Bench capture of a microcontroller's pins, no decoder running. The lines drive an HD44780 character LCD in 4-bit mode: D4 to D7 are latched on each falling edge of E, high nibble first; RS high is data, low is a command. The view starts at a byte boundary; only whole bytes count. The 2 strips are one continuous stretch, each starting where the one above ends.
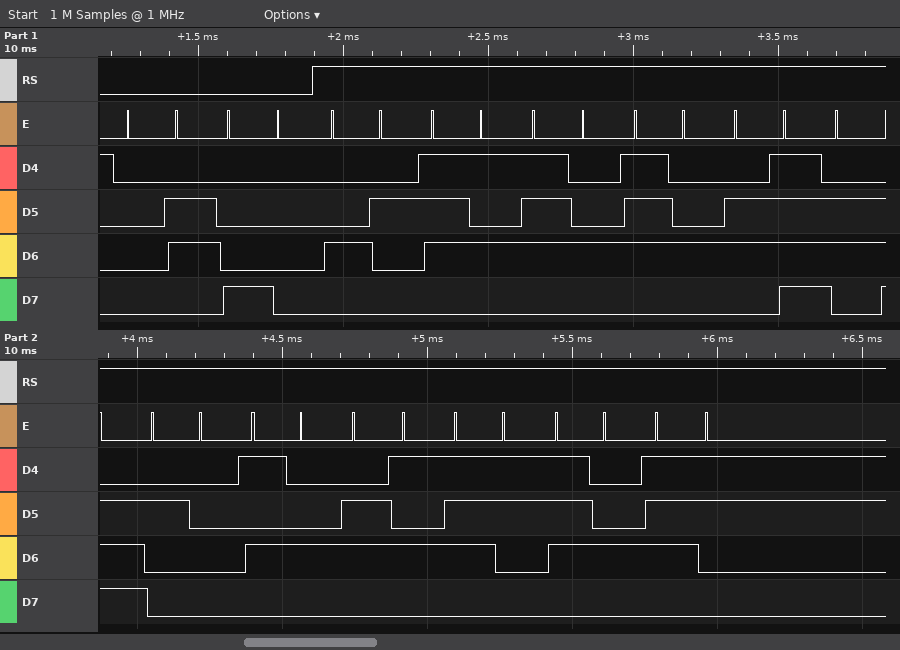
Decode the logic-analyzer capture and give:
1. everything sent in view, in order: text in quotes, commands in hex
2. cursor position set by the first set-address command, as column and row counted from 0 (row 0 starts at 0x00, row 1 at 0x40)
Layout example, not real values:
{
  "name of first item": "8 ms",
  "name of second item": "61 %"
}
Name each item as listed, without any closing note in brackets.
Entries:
{
  "everything sent in view, in order: text in quotes, commands in hex": "0x06 0x80 \"Button Tests\"",
  "cursor position set by the first set-address command, as column and row counted from 0": "column 0, row 0"
}
